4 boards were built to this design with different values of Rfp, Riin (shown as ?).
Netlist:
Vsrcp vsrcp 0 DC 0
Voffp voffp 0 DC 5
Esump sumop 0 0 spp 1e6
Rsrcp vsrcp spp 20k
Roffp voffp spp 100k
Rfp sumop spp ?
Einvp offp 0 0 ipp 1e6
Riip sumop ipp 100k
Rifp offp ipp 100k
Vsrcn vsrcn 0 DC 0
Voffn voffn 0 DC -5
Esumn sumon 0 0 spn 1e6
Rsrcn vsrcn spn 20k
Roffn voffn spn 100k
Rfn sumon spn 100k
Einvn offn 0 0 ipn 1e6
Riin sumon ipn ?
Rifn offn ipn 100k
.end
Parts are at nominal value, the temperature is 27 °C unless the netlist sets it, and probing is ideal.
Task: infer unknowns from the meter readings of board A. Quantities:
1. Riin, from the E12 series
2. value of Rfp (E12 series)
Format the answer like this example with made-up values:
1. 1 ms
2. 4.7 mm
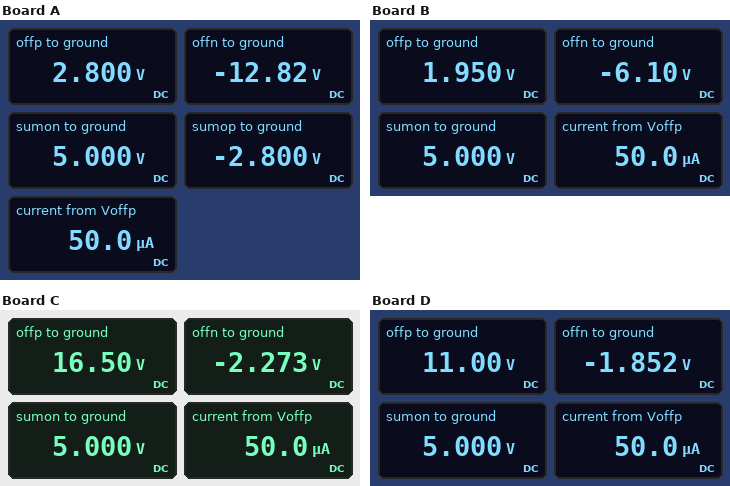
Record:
1. 39 kΩ
2. 56 kΩ
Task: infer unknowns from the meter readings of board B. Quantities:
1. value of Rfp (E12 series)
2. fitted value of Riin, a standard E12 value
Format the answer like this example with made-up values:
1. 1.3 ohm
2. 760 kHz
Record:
1. 39 kΩ
2. 82 kΩ
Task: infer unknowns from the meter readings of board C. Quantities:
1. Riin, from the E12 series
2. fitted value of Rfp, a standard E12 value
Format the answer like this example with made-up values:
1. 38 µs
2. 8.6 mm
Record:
1. 220 kΩ
2. 330 kΩ
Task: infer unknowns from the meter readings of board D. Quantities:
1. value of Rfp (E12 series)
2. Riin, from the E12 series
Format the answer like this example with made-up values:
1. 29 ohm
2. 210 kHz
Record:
1. 220 kΩ
2. 270 kΩ
